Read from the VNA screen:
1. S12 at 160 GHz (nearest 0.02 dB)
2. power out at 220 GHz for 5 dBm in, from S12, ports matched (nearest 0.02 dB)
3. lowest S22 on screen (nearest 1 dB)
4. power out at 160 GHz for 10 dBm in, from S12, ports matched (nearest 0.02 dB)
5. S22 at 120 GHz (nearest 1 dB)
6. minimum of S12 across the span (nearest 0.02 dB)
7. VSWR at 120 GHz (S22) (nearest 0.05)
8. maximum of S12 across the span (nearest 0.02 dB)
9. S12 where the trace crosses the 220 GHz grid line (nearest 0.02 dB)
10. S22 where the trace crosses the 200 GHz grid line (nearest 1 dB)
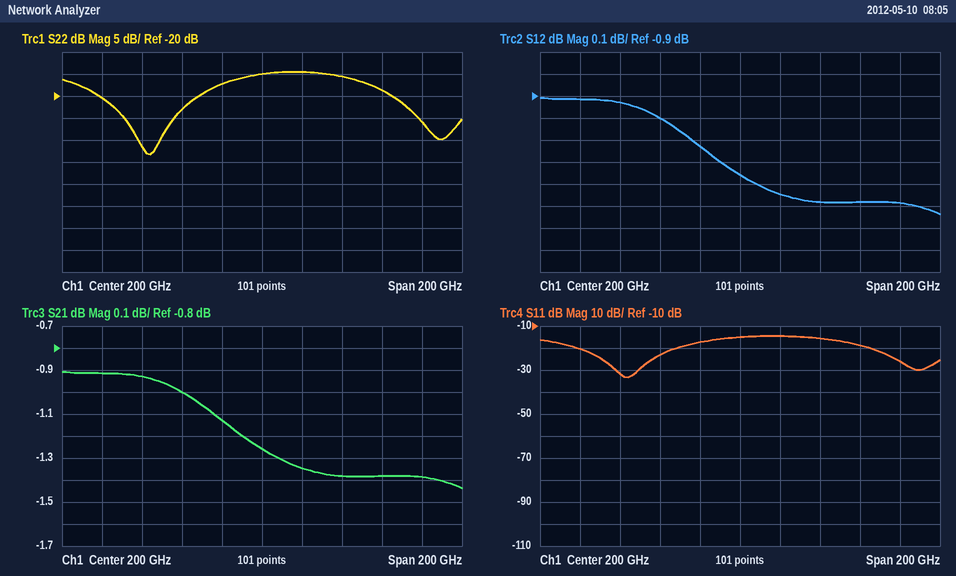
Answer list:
-1.00 dB
3.66 dBm
-33 dB
9.00 dBm
-20 dB
-1.44 dB
1.20
-0.90 dB
-1.34 dB
-15 dB
